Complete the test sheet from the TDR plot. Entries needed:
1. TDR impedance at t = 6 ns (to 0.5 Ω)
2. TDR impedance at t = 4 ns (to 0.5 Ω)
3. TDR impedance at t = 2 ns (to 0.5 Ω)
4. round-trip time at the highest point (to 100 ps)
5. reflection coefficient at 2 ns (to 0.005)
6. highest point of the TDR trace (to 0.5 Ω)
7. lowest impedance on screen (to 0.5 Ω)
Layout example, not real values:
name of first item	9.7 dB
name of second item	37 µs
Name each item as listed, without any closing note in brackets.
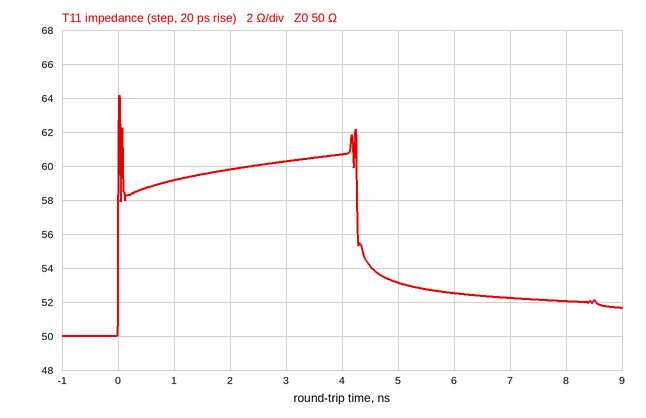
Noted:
TDR impedance at t = 6 ns	52.5 Ω
TDR impedance at t = 4 ns	60.5 Ω
TDR impedance at t = 2 ns	60.0 Ω
round-trip time at the highest point	0.0 ns
reflection coefficient at 2 ns	+0.090
highest point of the TDR trace	64.0 Ω
lowest impedance on screen	50.0 Ω
